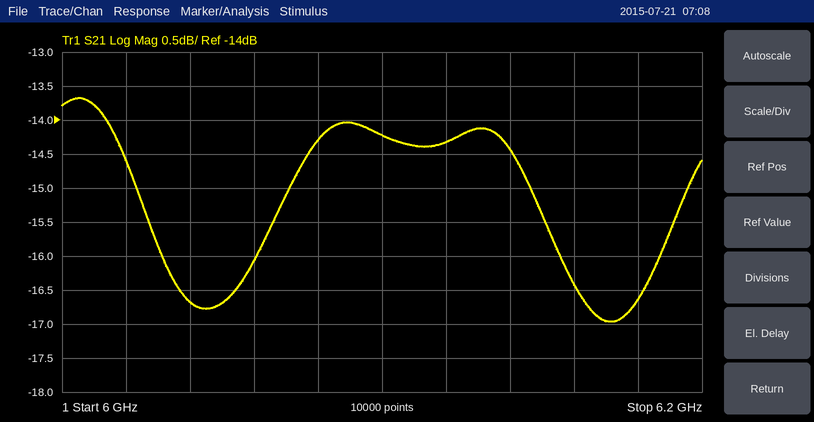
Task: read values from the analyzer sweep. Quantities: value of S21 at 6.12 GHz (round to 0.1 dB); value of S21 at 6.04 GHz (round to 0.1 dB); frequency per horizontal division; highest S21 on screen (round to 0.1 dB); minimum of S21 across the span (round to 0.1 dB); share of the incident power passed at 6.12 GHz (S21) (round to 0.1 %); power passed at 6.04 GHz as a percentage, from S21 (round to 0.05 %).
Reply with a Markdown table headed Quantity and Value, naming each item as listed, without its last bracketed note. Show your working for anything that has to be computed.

| Quantity | Value |
|---|---|
| value of S21 at 6.12 GHz | -14.3 dB |
| value of S21 at 6.04 GHz | -16.7 dB |
| frequency per horizontal division | 20 MHz |
| highest S21 on screen | -13.7 dB |
| minimum of S21 across the span | -17.0 dB |
| share of the incident power passed at 6.12 GHz (S21) | 10^(-14.3/10) ≈ 3.7 % |
| power passed at 6.04 GHz as a percentage, from S21 | 10^(-16.7/10) ≈ 2.14 %, so 2.15 % to the nearest 0.05 % |
